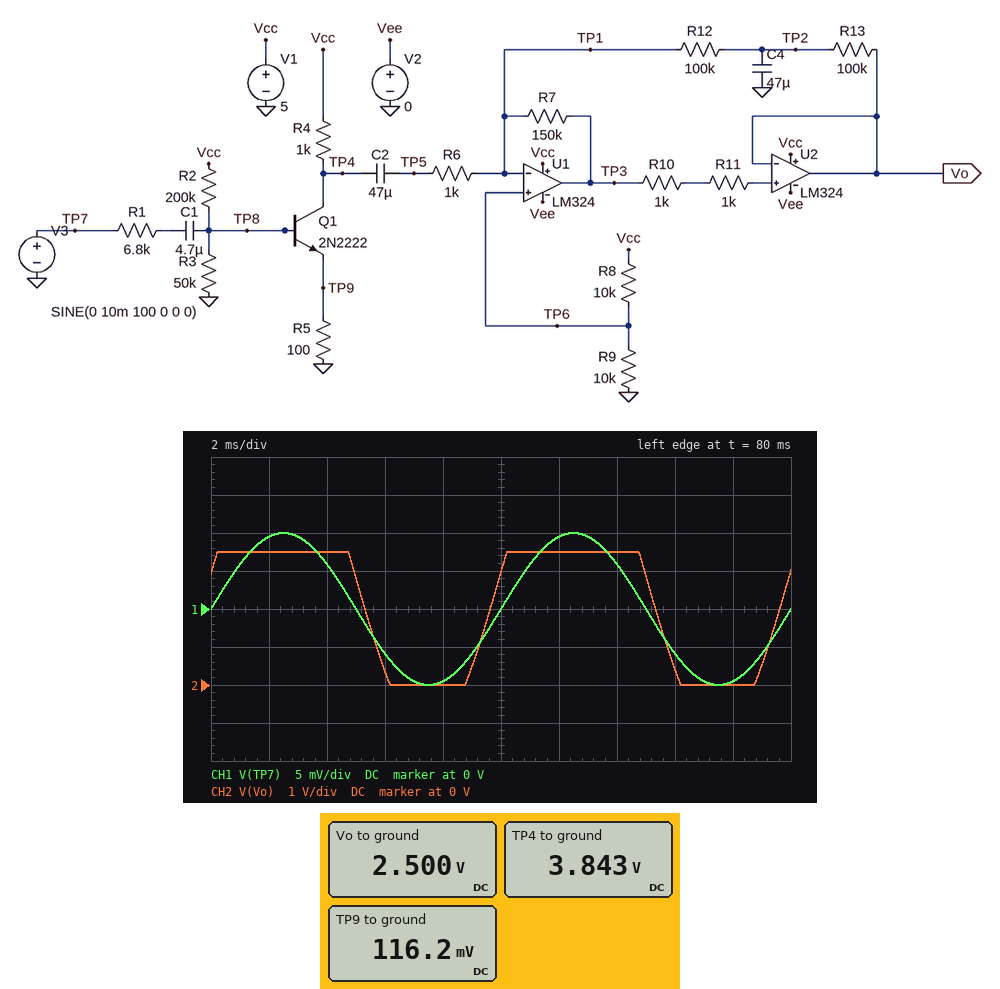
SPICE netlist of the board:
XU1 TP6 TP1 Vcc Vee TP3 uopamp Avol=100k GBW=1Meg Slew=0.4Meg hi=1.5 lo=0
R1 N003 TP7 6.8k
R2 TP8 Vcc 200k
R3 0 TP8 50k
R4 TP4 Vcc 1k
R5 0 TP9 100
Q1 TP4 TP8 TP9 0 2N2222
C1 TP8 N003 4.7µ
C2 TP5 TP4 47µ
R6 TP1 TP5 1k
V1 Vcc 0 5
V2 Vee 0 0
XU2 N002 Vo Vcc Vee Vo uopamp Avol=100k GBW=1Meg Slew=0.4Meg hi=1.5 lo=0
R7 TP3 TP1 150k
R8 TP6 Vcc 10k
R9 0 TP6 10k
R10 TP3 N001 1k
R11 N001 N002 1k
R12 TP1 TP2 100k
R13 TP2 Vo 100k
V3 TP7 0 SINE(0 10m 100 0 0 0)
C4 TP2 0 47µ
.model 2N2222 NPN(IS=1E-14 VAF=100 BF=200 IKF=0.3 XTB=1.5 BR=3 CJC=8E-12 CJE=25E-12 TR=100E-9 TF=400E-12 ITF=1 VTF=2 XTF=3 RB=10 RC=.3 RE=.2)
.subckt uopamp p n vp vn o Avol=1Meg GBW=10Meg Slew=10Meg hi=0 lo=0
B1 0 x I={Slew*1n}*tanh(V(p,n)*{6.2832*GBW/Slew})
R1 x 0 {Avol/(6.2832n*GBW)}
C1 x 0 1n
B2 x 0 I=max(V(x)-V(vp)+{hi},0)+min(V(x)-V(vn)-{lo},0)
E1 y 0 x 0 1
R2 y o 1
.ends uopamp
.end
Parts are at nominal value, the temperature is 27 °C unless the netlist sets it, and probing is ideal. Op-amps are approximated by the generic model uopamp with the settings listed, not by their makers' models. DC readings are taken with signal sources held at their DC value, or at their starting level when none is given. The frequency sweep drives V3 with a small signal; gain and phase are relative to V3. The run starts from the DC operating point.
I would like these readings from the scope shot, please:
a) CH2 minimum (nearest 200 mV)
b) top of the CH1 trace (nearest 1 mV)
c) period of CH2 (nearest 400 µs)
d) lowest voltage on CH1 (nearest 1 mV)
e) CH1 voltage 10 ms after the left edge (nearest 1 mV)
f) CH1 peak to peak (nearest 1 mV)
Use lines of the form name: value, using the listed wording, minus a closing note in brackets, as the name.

CH2 minimum: 0 V
top of the CH1 trace: 10 mV
period of CH2: 10.0 ms
lowest voltage on CH1: -10 mV
CH1 voltage 10 ms after the left edge: 0 V
CH1 peak to peak: 20 mV
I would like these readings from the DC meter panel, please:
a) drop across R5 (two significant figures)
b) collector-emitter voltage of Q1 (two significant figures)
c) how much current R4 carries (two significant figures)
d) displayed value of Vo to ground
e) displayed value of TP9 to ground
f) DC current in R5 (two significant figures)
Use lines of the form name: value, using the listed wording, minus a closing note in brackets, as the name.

drop across R5: 120 mV
collector-emitter voltage of Q1: 3.7 V
how much current R4 carries: 1.2 mA
displayed value of Vo to ground: 2.500 V
displayed value of TP9 to ground: 116.2 mV
DC current in R5: 1.2 mA
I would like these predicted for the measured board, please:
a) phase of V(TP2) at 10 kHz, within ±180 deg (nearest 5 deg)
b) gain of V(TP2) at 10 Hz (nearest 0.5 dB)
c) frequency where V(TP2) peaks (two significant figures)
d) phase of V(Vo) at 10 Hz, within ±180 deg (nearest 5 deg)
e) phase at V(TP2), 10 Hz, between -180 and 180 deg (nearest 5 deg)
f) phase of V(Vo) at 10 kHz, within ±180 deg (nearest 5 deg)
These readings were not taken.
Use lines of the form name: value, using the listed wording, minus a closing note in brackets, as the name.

phase of V(TP2) at 10 kHz, within ±180 deg: -130 deg
gain of V(TP2) at 10 Hz: 3.0 dB
frequency where V(TP2) peaks: 1.6 Hz
phase of V(Vo) at 10 Hz, within ±180 deg: 20 deg
phase at V(TP2), 10 Hz, between -180 and 180 deg: -70 deg
phase of V(Vo) at 10 kHz, within ±180 deg: -40 deg
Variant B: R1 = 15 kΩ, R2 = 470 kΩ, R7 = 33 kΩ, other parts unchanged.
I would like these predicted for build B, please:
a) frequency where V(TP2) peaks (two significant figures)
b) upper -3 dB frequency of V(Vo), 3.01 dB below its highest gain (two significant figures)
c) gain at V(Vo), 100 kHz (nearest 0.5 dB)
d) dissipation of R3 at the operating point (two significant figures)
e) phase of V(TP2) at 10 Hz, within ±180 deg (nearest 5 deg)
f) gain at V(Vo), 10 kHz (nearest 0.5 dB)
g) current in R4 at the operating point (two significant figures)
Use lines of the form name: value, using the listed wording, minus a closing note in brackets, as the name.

frequency where V(TP2) peaks: 990 mHz
upper -3 dB frequency of V(Vo), 3.01 dB below its highest gain: 55 kHz
gain at V(Vo), 100 kHz: -11.5 dB
dissipation of R3 at the operating point: 4.6 µW
phase of V(TP2) at 10 Hz, within ±180 deg: -75 deg
gain at V(Vo), 10 kHz: -5.0 dB
current in R4 at the operating point: 1.2 µA
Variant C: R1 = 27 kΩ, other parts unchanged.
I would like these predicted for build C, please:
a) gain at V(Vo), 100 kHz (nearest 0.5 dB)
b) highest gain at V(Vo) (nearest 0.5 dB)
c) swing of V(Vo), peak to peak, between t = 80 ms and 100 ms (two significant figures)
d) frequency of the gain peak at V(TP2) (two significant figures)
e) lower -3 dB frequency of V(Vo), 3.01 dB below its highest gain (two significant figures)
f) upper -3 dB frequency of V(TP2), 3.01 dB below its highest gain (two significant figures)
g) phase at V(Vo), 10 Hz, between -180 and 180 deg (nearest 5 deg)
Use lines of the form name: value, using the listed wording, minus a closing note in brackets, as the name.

gain at V(Vo), 100 kHz: 28.5 dB
highest gain at V(Vo): 47.0 dB
swing of V(Vo), peak to peak, between t = 80 ms and 100 ms: 3.0 V
frequency of the gain peak at V(TP2): 1.2 Hz
lower -3 dB frequency of V(Vo), 3.01 dB below its highest gain: 2.0 Hz
upper -3 dB frequency of V(TP2), 3.01 dB below its highest gain: 3.0 Hz
phase at V(Vo), 10 Hz, between -180 and 180 deg: 15 deg
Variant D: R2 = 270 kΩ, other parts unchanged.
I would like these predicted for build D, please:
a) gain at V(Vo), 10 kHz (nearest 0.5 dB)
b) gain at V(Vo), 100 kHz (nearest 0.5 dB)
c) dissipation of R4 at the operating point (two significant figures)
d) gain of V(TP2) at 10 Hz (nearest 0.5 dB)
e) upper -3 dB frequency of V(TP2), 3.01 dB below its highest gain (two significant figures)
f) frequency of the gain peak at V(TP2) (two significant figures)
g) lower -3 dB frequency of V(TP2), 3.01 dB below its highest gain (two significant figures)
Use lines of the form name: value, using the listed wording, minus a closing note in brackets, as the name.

gain at V(Vo), 10 kHz: 49.0 dB
gain at V(Vo), 100 kHz: 33.0 dB
dissipation of R4 at the operating point: 230 µW
gain of V(TP2) at 10 Hz: 1.5 dB
upper -3 dB frequency of V(TP2), 3.01 dB below its highest gain: 3.7 Hz
frequency of the gain peak at V(TP2): 1.5 Hz
lower -3 dB frequency of V(TP2), 3.01 dB below its highest gain: 640 mHz
